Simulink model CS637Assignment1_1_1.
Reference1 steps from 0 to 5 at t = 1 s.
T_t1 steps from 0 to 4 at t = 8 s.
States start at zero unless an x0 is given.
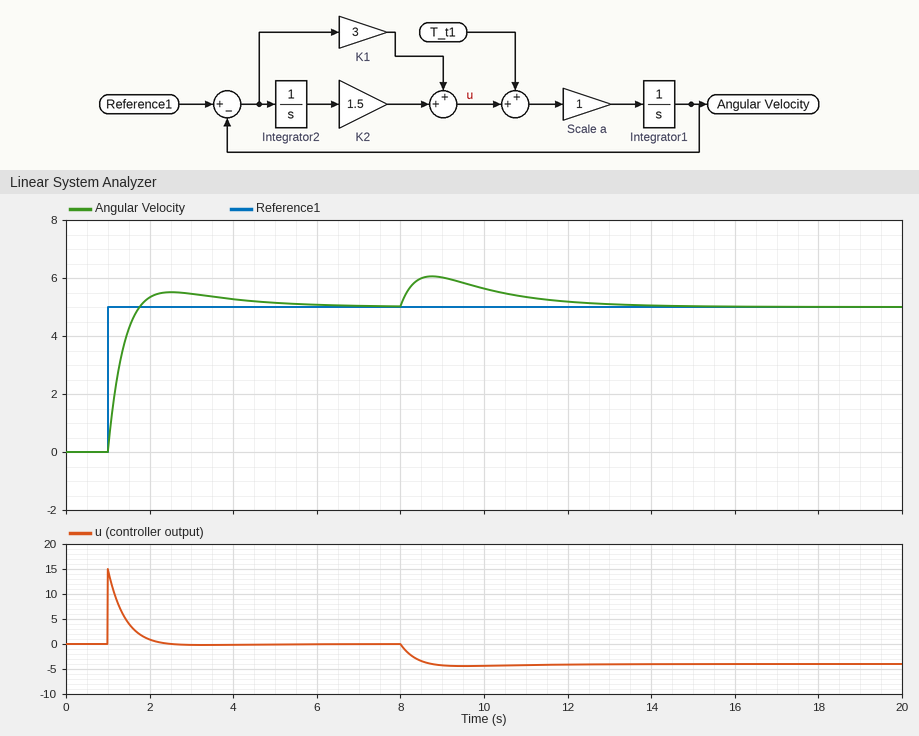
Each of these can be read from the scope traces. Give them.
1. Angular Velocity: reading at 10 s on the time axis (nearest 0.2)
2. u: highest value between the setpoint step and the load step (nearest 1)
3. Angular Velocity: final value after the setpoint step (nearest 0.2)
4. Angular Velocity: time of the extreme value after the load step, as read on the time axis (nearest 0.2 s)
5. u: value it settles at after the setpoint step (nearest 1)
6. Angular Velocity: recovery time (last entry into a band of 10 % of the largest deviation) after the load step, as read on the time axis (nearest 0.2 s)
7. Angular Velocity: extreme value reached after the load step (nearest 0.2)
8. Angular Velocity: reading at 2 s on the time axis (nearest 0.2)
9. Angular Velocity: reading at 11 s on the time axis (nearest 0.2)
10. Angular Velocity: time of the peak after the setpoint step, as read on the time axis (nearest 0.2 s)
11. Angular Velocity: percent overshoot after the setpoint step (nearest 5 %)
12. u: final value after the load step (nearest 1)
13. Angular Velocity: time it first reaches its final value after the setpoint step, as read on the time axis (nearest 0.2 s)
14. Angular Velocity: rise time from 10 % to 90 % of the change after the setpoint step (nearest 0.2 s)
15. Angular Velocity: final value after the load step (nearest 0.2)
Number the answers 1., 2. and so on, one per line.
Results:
1. 5.6
2. 15
3. 5.0
4. 8.8 s
5. 0
6. 13.0 s
7. 6.0
8. 5.4
9. 5.4
10. 2.6 s
11. 10 %
12. -4
13. 1.8 s
14. 0.6 s
15. 5.0
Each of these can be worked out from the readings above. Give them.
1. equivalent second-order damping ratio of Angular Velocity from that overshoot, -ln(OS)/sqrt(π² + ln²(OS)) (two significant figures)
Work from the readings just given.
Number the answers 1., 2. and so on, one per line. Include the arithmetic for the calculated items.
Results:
1. ln(0.1) = -2.303; 2.303 / sqrt(9.870 + 5.302) = 0.59
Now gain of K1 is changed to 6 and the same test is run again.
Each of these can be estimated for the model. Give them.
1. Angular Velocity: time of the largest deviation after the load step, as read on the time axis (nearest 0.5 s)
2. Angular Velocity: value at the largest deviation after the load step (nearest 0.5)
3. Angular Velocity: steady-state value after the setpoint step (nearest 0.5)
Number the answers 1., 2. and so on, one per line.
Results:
1. 8.5 s
2. 5.5
3. 5.0
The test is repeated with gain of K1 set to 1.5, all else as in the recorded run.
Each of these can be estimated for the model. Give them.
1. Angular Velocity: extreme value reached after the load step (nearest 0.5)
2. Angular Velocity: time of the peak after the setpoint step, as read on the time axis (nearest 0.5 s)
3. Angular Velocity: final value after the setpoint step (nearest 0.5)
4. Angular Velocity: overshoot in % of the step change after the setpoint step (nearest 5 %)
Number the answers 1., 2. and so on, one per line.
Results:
1. 6.5
2. 3.0 s
3. 5.0
4. 25 %
